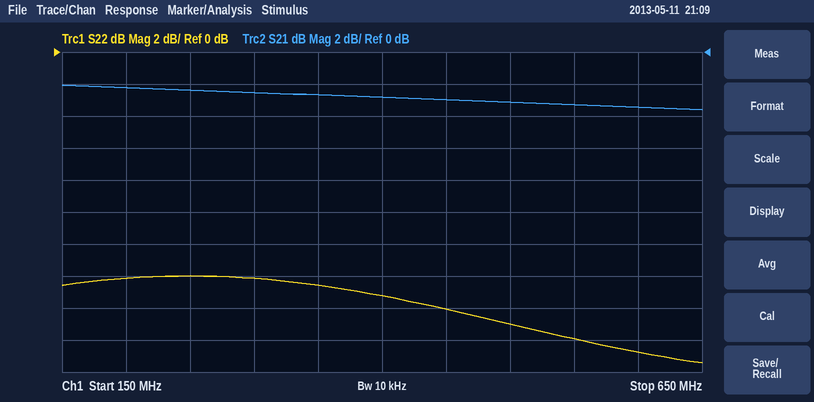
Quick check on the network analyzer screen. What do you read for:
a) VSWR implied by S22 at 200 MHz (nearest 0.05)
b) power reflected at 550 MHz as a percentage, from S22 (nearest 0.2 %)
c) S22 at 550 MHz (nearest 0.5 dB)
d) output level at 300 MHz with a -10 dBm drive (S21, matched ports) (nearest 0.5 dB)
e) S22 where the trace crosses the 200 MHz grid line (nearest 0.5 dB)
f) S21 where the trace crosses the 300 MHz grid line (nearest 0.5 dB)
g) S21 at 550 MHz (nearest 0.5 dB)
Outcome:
1.50
1.6 %
-18.0 dB
-12.5 dBm
-14.0 dB
-2.5 dB
-3.5 dB
